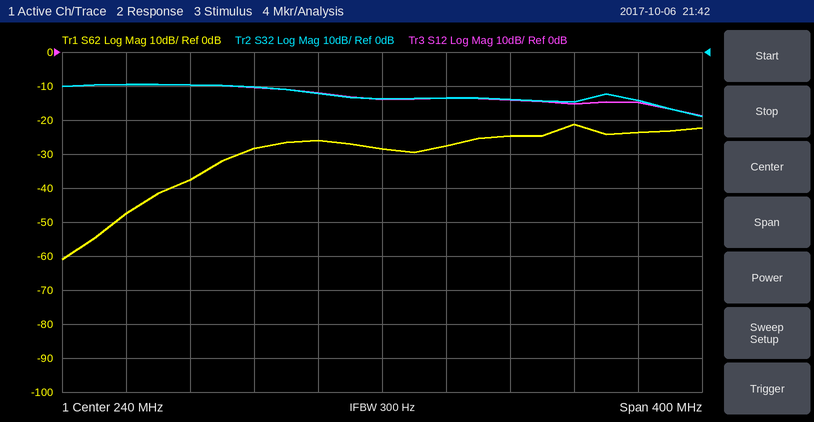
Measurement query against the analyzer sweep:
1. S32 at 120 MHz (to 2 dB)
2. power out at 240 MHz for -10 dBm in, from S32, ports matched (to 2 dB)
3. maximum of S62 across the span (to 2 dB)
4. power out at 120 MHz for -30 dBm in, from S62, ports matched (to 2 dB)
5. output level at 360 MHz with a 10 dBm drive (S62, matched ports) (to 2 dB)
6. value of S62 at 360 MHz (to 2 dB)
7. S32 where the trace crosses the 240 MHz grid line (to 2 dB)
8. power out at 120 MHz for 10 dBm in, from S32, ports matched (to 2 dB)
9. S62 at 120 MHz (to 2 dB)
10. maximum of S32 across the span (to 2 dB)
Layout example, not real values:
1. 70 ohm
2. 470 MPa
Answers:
1. -10 dB
2. -24 dBm
3. -22 dB
4. -68 dBm
5. -12 dBm
6. -22 dB
7. -14 dB
8. 0 dBm
9. -38 dB
10. -10 dB
